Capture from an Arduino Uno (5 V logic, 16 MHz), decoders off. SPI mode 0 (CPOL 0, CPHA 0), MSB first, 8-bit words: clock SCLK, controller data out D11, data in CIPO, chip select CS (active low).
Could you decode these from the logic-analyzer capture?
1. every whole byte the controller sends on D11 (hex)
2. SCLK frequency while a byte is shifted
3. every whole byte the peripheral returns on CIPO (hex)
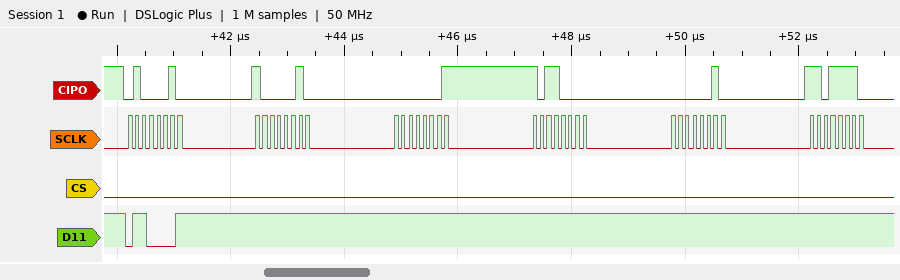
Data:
61 FF FF FF FF FF
8 MHz
42 82 01 B0 02 DE
